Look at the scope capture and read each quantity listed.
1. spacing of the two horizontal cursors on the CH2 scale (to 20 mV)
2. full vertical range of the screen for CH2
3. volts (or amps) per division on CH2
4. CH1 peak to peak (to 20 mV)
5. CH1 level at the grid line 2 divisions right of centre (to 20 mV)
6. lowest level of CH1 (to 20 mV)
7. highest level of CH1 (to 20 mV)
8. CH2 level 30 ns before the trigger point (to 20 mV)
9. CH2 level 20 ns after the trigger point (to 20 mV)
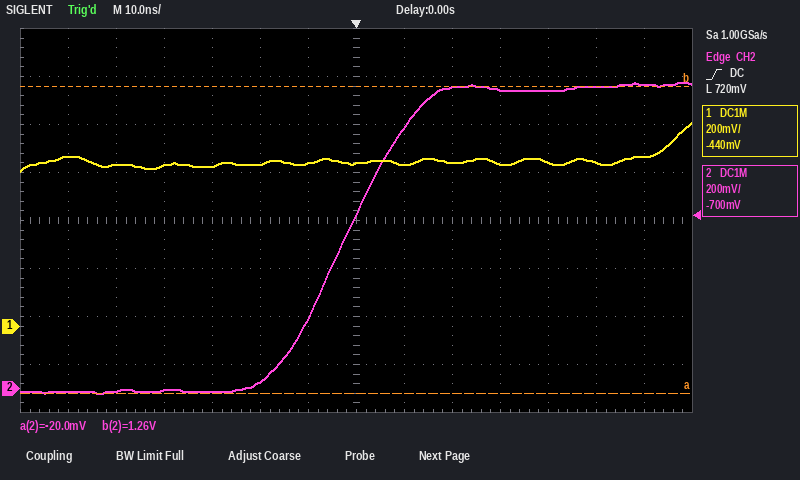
1.28 V
1.6 V
200 mV
200 mV
680 mV
640 mV
840 mV
-20 mV
1.26 V
